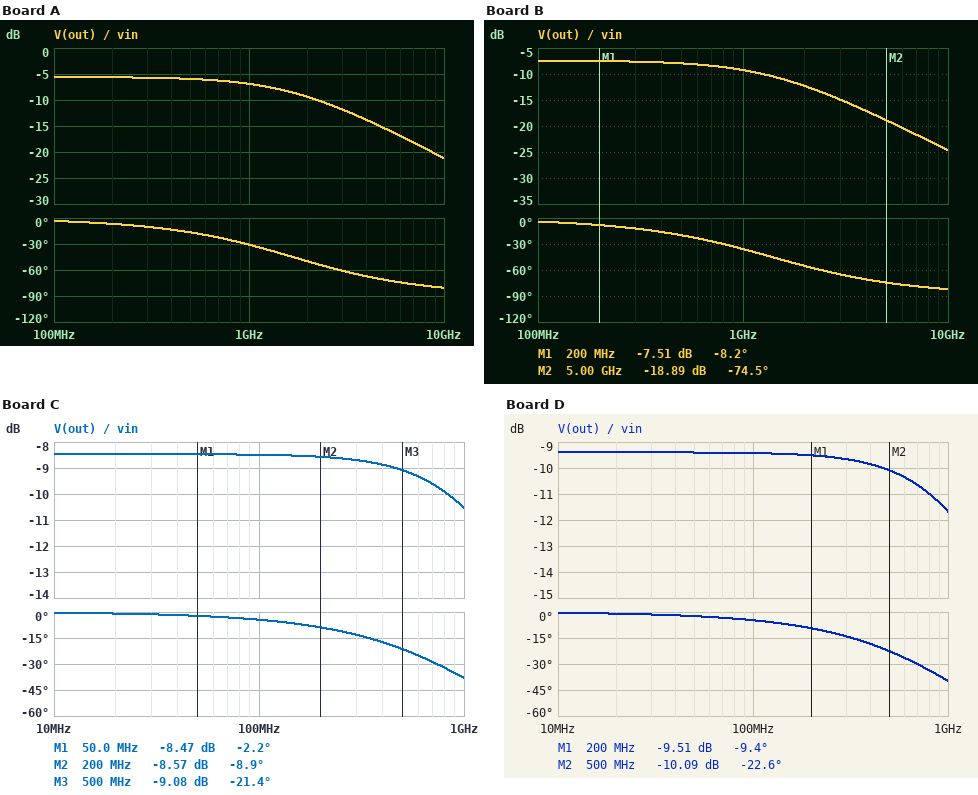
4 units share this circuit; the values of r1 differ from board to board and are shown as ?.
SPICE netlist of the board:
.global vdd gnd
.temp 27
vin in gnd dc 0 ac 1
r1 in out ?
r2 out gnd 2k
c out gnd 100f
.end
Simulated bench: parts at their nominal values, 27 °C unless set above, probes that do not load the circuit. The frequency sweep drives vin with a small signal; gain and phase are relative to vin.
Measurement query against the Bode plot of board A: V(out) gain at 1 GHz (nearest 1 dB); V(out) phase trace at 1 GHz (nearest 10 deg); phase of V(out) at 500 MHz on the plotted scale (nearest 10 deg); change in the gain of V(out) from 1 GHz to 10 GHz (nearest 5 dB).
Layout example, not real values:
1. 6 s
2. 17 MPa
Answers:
1. -7 dB
2. -30 deg
3. -20 deg
4. -15 dB
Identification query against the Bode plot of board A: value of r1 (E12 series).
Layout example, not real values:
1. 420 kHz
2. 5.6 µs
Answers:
1. 1.8 kΩ
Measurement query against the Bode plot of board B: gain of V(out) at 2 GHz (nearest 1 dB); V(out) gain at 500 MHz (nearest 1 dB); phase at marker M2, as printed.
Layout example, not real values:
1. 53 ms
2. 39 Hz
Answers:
1. -12 dB
2. -8 dB
3. -74.5 deg
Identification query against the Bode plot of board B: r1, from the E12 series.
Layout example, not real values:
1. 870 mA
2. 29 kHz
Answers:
1. 2.7 kΩ
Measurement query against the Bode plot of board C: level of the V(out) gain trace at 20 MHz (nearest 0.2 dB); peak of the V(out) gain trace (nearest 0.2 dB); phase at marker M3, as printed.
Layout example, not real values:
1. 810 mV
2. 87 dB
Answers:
1. -8.4 dB
2. -8.4 dB
3. -21.4 deg
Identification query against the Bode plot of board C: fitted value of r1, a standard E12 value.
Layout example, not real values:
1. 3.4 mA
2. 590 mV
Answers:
1. 3.3 kΩ
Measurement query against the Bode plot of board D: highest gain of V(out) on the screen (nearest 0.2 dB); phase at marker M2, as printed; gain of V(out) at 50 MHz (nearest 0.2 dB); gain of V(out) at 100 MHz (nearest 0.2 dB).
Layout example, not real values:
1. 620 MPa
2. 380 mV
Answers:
1. -9.4 dB
2. -22.6 deg
3. -9.4 dB
4. -9.4 dB
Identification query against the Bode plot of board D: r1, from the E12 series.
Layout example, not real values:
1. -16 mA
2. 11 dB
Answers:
1. 3.9 kΩ
